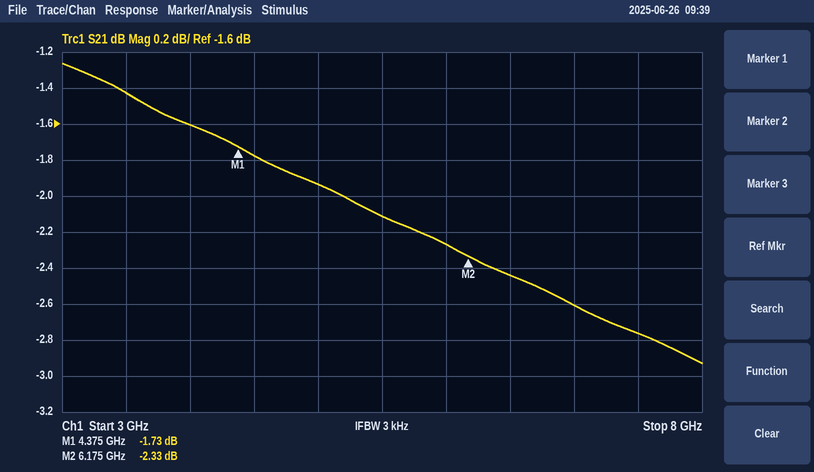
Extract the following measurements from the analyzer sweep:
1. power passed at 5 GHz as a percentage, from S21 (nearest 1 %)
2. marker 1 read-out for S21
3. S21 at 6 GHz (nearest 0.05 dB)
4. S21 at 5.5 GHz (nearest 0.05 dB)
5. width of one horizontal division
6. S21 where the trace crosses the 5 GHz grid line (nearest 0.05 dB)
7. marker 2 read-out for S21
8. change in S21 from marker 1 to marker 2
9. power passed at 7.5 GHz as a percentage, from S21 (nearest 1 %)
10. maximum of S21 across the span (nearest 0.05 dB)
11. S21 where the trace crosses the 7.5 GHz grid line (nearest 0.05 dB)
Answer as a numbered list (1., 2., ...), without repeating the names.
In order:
1. 64 %
2. -1.73 dB
3. -2.25 dB
4. -2.10 dB
5. 500 MHz
6. -1.95 dB
7. -2.33 dB
8. -0.60 dB
9. 53 %
10. -1.25 dB
11. -2.75 dB
